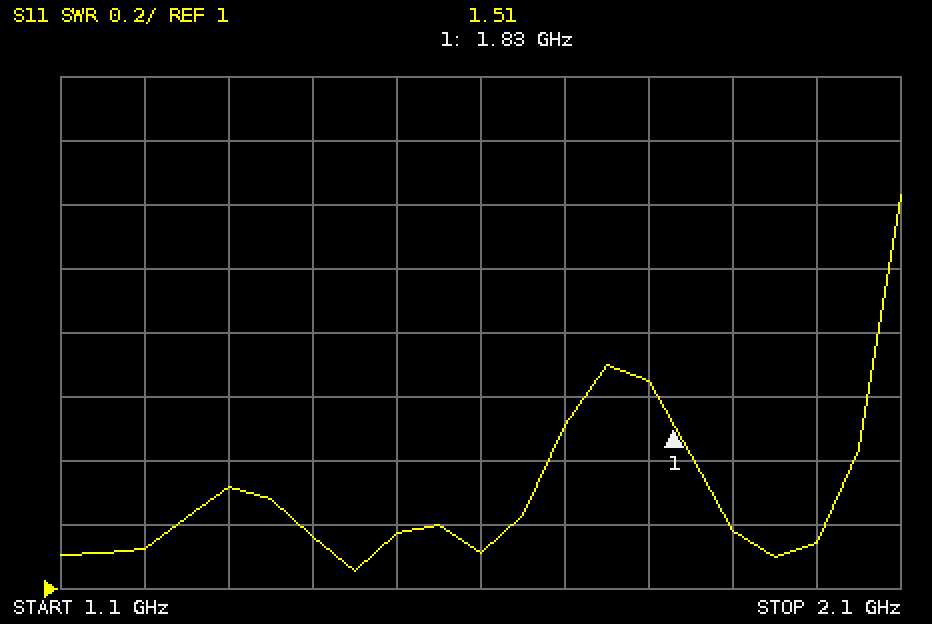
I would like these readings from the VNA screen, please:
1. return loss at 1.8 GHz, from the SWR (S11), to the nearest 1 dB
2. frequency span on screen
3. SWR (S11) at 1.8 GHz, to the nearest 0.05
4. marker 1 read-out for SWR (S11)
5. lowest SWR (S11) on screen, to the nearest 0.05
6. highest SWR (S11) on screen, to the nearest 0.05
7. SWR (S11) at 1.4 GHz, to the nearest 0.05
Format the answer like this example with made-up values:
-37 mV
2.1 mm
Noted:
12 dB
1 GHz
1.65
1.51
1.05
2.25
1.15
